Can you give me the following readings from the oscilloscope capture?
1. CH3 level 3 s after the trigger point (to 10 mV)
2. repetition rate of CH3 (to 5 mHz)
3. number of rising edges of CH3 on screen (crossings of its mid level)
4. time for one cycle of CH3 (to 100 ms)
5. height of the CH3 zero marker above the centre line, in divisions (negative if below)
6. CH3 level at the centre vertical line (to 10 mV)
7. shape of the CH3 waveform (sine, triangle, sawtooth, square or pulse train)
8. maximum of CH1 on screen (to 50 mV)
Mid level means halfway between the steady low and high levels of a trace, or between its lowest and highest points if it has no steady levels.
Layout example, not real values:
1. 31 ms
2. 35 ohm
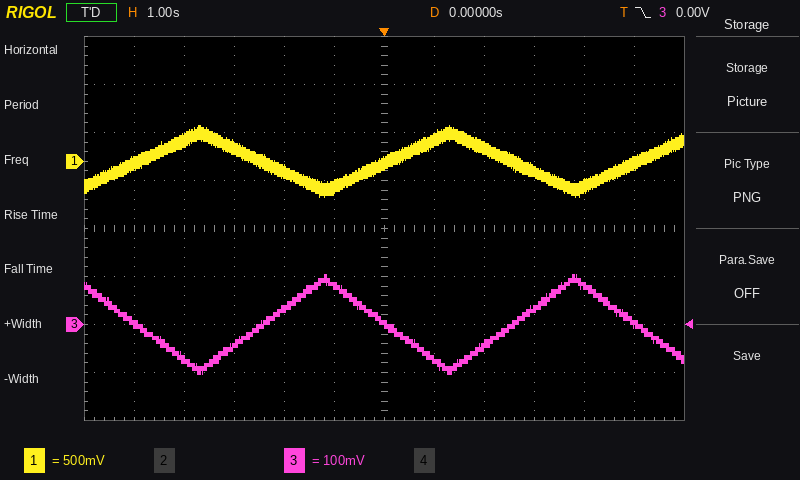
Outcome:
1. 30 mV
2. 200 mHz
3. 2
4. 5.0 s
5. -2.0 div
6. 0 mV
7. triangle
8. 350 mV
